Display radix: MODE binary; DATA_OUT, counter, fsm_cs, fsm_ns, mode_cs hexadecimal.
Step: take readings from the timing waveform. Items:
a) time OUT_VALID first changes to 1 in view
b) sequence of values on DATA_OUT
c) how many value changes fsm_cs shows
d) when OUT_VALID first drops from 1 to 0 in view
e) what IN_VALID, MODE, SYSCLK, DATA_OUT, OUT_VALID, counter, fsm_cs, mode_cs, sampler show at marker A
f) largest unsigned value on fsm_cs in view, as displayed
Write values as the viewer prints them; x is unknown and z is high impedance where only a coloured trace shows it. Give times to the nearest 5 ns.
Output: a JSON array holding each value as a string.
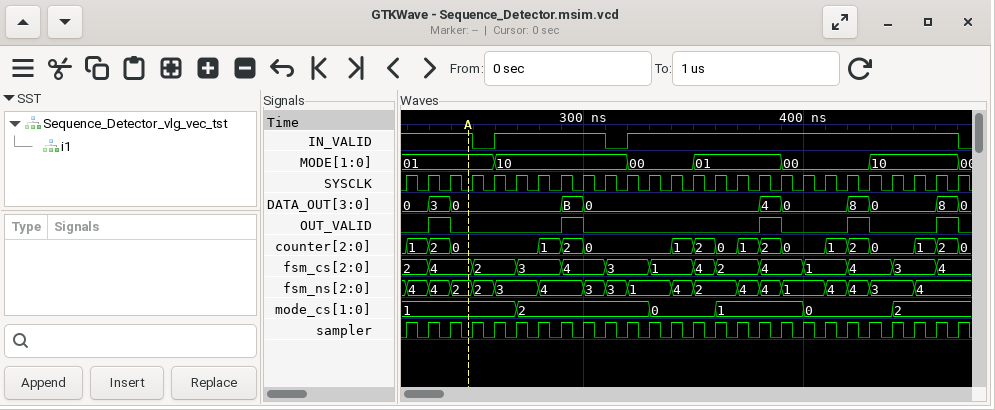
["230 ns", "0, 3, 0, B, 0, 4, 0, 8, 0, 8, 0", "13", "240 ns", "IN_VALID=1, MODE=01, SYSCLK=0, DATA_OUT=0, OUT_VALID=0, counter=0, fsm_cs=4, mode_cs=1, sampler=0", "4"]
